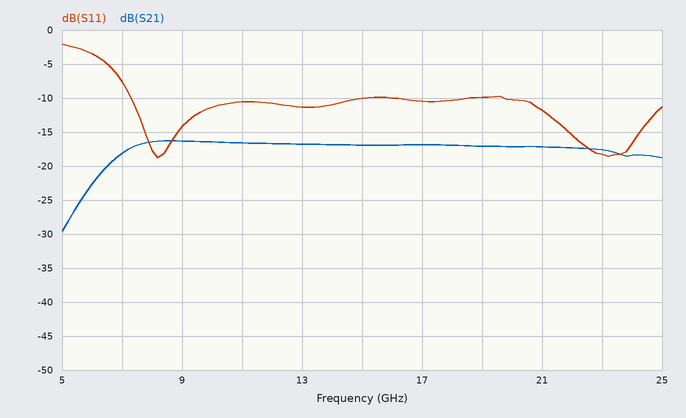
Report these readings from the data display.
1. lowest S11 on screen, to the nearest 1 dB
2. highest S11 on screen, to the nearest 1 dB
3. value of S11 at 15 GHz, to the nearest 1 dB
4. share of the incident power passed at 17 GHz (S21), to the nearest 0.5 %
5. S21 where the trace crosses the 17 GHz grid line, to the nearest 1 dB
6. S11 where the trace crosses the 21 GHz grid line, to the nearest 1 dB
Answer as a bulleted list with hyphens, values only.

- -19 dB
- -2 dB
- -10 dB
- 2.0 %
- -17 dB
- -12 dB
